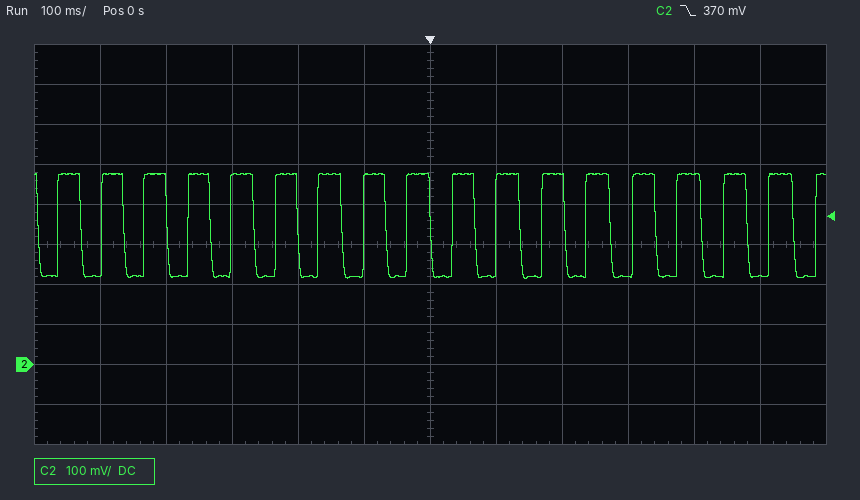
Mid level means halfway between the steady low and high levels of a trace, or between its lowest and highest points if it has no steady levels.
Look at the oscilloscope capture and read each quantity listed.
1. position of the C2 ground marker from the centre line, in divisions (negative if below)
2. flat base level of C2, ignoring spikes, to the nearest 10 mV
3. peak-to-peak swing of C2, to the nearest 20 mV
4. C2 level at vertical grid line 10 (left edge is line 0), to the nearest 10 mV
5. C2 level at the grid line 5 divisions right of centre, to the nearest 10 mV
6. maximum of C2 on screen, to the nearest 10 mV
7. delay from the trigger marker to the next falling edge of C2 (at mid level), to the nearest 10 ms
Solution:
-3.0 div
220 mV
260 mV
480 mV
220 mV
480 mV
70 ms
